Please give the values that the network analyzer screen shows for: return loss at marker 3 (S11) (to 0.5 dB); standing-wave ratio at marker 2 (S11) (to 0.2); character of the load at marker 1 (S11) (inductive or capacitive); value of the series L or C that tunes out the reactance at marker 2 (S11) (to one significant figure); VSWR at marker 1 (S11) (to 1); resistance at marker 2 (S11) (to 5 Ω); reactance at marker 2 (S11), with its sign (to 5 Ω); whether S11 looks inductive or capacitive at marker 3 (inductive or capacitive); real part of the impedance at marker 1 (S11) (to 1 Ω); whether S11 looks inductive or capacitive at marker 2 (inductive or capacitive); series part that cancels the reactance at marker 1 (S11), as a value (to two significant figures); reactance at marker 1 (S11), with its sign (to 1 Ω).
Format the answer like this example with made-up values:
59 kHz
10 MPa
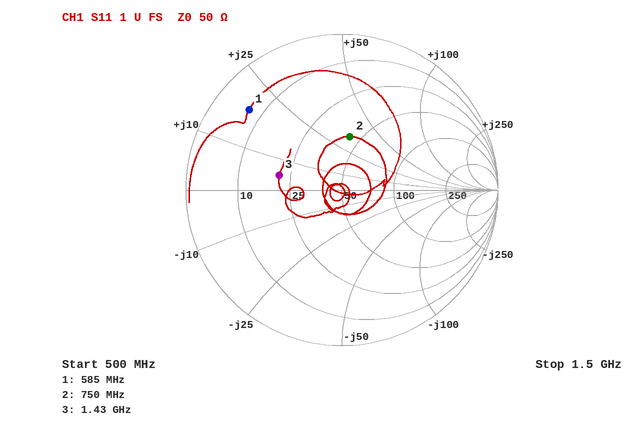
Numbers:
7.5 dB
2.0
inductive
6 pF
8
45 Ω
+35 Ω
inductive
7 Ω
inductive
15 pF
+18 Ω
